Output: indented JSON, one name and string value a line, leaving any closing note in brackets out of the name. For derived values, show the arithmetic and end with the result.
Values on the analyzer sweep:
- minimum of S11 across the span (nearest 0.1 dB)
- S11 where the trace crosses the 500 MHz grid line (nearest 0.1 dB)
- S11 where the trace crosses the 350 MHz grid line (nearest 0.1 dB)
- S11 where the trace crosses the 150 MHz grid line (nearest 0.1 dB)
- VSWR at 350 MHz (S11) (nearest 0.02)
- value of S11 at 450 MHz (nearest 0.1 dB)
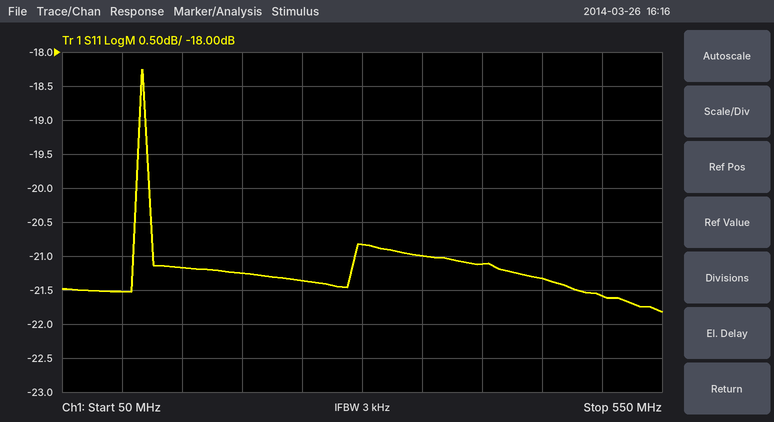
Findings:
{
  "minimum of S11 across the span": "-21.8 dB",
  "S11 where the trace crosses the 500 MHz grid line": "-21.6 dB",
  "S11 where the trace crosses the 350 MHz grid line": "-21.0 dB",
  "S11 where the trace crosses the 150 MHz grid line": "-21.2 dB",
  "VSWR at 350 MHz (S11)": "|Γ| = 10^(-21/20) = 0.0891; VSWR = (1 + 0.0891)/(1 − 0.0891) ≈ 1.20",
  "value of S11 at 450 MHz": "-21.3 dB"
}
